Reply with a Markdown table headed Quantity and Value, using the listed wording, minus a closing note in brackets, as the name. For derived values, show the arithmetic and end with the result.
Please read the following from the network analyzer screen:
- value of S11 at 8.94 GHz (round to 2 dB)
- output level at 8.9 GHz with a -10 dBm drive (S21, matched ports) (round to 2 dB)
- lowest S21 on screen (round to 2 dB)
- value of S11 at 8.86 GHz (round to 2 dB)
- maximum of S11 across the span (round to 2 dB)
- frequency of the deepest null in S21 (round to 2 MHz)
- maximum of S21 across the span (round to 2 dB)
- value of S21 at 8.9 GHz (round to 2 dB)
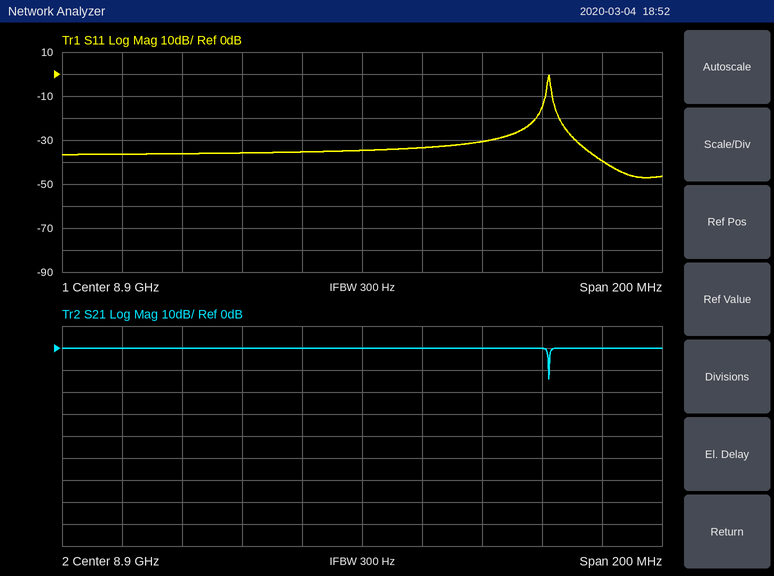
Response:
| Quantity | Value |
|---|---|
| value of S11 at 8.94 GHz | -30 dB |
| output level at 8.9 GHz with a -10 dBm drive (S21, matched ports) | -10 dBm + (0 dB) = -10 dBm |
| lowest S21 on screen | -14 dB |
| value of S11 at 8.86 GHz | -36 dB |
| maximum of S11 across the span | 0 dB |
| frequency of the deepest null in S21 | 8.962 GHz |
| maximum of S21 across the span | 0 dB |
| value of S21 at 8.9 GHz | 0 dB |
